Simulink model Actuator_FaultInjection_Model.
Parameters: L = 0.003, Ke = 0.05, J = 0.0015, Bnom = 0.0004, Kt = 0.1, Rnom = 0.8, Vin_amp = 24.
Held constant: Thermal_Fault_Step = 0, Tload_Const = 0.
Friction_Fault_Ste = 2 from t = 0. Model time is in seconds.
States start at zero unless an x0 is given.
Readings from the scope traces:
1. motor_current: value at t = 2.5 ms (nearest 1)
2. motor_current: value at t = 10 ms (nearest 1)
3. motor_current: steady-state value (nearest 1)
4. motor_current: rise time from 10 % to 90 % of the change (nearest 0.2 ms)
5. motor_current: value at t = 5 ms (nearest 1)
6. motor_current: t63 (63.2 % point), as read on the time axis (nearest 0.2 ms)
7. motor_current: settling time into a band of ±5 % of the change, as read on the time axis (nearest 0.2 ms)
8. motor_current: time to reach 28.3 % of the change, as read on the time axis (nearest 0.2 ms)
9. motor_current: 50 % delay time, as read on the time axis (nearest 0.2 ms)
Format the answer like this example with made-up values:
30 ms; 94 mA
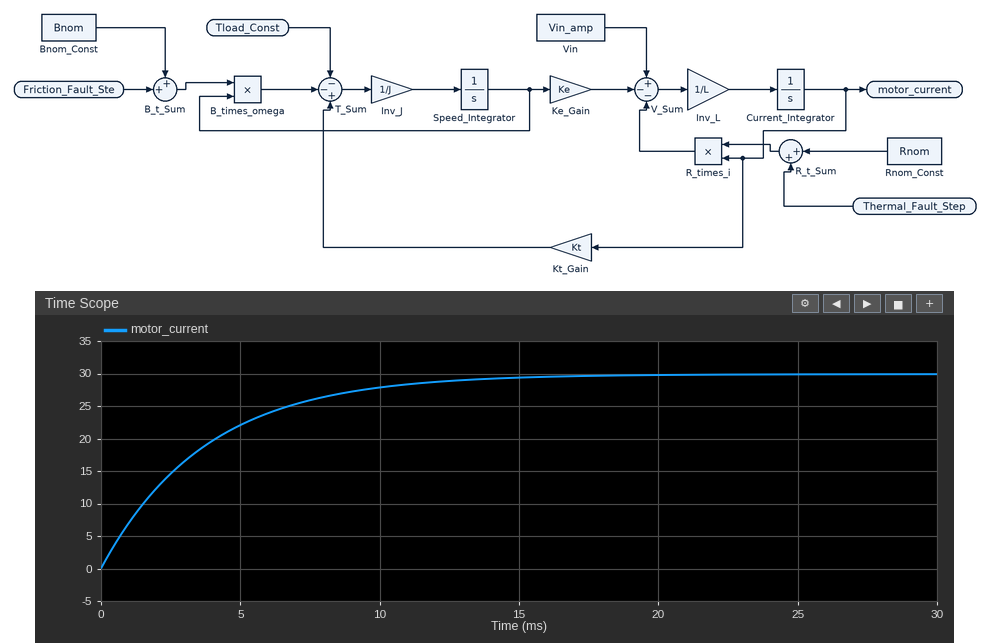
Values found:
15; 28; 30; 8.2 ms; 22; 3.8 ms; 11.2 ms; 1.2 ms; 2.6 ms
